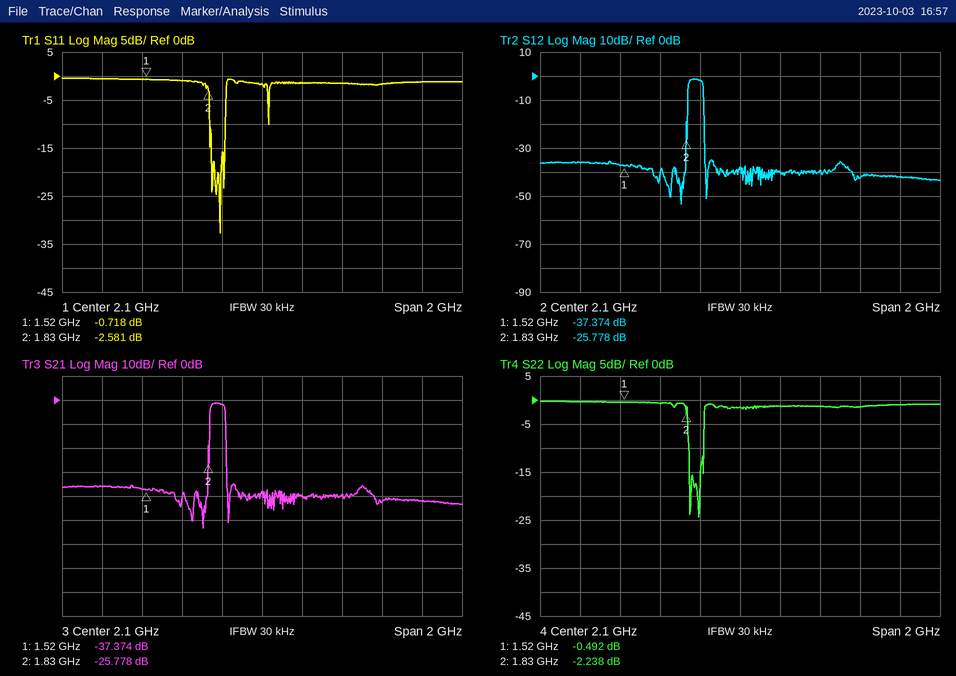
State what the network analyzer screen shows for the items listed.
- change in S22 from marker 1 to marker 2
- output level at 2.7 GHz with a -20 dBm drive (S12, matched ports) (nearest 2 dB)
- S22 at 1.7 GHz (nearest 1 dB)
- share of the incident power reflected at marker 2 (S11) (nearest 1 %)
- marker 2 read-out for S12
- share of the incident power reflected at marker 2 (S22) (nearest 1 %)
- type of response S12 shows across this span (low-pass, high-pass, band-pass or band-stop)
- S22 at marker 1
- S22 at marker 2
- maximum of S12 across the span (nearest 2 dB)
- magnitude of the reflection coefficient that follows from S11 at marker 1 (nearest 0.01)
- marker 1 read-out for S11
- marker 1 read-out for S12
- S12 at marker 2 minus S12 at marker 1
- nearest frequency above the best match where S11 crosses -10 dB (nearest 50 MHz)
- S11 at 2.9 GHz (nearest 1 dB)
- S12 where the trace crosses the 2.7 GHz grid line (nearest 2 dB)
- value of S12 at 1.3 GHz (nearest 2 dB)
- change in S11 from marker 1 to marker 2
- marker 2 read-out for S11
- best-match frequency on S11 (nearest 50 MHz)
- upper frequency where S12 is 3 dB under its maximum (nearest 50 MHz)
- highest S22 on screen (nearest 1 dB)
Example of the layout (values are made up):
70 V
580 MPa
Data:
-1.746 dB
-62 dBm
-1 dB
55 %
-25.778 dB
60 %
band-pass
-0.492 dB
-2.238 dB
-2 dB
0.92
-0.718 dB
-37.374 dB
11.596 dB
1.90 GHz
-1 dB
-42 dB
-36 dB
-1.863 dB
-2.581 dB
1.90 GHz
1.90 GHz
0 dB
